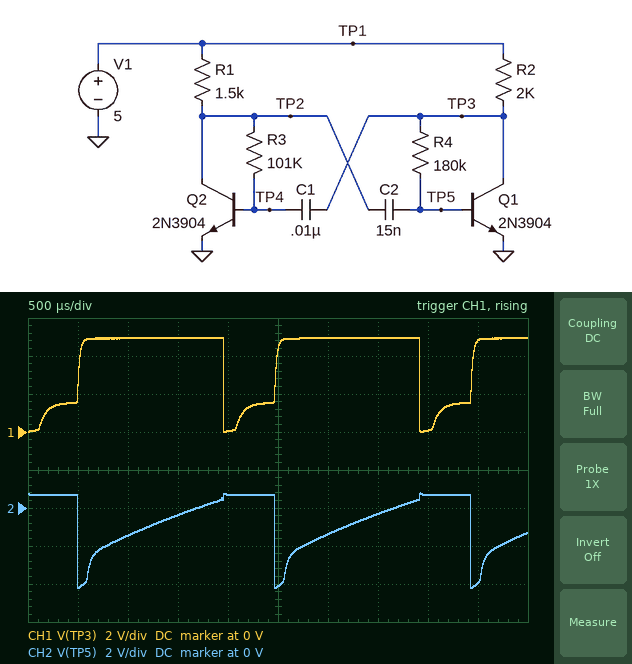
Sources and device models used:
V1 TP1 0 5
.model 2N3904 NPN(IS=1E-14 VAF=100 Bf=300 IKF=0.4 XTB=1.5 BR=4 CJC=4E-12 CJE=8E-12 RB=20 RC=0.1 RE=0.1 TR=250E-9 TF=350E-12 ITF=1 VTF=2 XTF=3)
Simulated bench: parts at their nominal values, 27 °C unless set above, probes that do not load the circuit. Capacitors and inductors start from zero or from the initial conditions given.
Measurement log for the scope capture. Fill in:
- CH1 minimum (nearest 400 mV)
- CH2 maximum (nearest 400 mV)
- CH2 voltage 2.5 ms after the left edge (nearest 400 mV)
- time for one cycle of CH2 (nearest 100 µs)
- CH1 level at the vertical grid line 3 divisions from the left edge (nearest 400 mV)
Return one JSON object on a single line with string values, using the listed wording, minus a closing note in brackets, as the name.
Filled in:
{"CH1 minimum": "0 V", "CH2 maximum": "800 mV", "CH2 voltage 2.5 ms after the left edge": "-4.0 V", "time for one cycle of CH2": "2.0 ms", "CH1 level at the vertical grid line 3 divisions from the left edge": "4.8 V"}
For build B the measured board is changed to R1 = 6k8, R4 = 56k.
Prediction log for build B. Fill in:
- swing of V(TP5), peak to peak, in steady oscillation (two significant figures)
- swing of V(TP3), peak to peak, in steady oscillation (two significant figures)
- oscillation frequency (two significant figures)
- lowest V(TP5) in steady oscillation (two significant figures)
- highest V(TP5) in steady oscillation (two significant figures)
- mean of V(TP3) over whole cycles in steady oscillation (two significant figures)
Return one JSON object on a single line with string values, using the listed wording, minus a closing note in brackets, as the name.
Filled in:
{"swing of V(TP5), peak to peak, in steady oscillation": "4.7 V", "swing of V(TP3), peak to peak, in steady oscillation": "4.8 V", "oscillation frequency": "840 Hz", "lowest V(TP5) in steady oscillation": "-4.0 V", "highest V(TP5) in steady oscillation": "710 mV", "mean of V(TP3) over whole cycles in steady oscillation": "2.2 V"}
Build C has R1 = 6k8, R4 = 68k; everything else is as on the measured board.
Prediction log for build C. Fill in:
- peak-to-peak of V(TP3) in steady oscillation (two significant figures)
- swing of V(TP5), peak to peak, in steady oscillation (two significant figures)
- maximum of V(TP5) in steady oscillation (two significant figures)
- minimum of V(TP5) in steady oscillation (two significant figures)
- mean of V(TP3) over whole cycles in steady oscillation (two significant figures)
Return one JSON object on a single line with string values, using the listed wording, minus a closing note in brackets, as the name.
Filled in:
{"peak-to-peak of V(TP3) in steady oscillation": "4.8 V", "swing of V(TP5), peak to peak, in steady oscillation": "4.7 V", "maximum of V(TP5) in steady oscillation": "710 mV", "minimum of V(TP5) in steady oscillation": "-4.0 V", "mean of V(TP3) over whole cycles in steady oscillation": "2.4 V"}
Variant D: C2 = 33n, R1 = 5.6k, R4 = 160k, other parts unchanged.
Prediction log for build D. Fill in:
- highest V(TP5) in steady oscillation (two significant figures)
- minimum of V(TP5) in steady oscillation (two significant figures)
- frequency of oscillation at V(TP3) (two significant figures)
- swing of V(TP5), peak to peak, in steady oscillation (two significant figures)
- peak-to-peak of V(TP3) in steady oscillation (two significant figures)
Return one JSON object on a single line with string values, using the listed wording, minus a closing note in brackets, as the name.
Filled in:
{"highest V(TP5) in steady oscillation": "710 mV", "minimum of V(TP5) in steady oscillation": "-4.0 V", "frequency of oscillation at V(TP3)": "260 Hz", "swing of V(TP5), peak to peak, in steady oscillation": "4.7 V", "peak-to-peak of V(TP3) in steady oscillation": "4.9 V"}
